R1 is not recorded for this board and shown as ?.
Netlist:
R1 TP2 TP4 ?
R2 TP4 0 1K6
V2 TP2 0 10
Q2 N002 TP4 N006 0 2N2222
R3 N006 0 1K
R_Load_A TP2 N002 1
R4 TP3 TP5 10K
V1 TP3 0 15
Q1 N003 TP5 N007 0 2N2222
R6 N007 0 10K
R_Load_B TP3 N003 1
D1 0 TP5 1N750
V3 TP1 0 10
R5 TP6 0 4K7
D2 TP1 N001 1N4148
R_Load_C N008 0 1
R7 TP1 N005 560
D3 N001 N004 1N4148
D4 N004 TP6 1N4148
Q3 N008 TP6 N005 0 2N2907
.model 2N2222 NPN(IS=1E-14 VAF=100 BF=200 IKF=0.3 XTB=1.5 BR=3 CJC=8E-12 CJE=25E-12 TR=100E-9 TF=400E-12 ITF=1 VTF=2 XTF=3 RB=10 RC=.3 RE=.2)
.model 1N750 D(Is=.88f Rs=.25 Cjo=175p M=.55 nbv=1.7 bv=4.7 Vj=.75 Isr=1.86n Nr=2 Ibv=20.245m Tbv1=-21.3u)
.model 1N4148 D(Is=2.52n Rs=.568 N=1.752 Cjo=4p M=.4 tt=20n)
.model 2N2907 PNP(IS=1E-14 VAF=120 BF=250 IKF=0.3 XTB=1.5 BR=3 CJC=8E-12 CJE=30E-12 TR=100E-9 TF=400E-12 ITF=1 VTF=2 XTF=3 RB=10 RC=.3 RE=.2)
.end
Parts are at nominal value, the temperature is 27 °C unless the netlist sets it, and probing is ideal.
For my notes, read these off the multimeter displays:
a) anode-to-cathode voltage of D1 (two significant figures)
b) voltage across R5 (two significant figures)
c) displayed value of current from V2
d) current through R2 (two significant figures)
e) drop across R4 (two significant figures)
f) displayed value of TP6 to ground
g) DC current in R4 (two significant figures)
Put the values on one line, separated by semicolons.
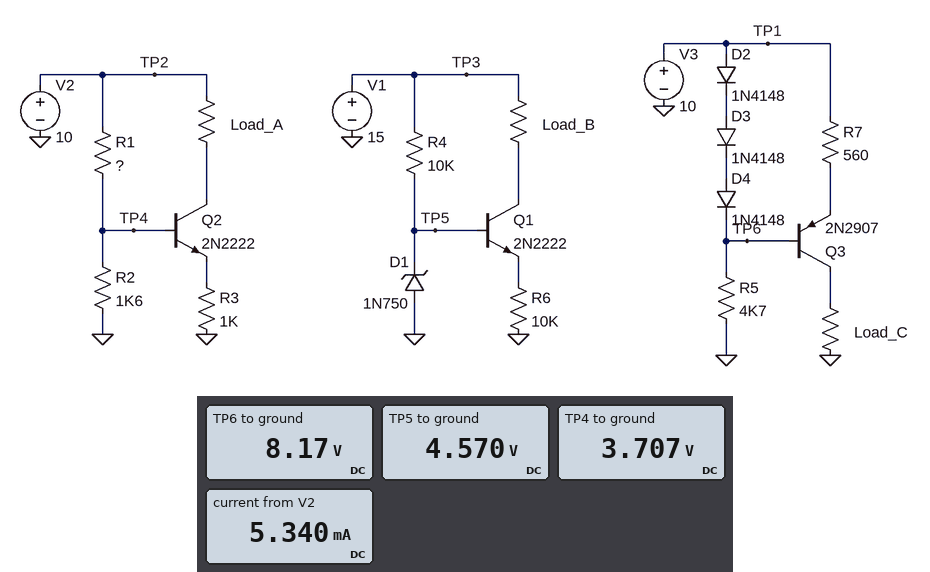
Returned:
-4.6 V; 8.2 V; 5.340 mA; 2.3 mA; 10 V; 8.17 V; 1.0 mA
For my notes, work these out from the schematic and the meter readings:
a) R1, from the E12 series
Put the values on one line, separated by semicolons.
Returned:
2.7 kΩ
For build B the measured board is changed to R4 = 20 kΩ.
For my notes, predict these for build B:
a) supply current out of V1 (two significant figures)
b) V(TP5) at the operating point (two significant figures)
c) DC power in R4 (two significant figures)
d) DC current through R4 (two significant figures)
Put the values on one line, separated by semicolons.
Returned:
910 µA; 4.5 V; 5.5 mW; 520 µA
